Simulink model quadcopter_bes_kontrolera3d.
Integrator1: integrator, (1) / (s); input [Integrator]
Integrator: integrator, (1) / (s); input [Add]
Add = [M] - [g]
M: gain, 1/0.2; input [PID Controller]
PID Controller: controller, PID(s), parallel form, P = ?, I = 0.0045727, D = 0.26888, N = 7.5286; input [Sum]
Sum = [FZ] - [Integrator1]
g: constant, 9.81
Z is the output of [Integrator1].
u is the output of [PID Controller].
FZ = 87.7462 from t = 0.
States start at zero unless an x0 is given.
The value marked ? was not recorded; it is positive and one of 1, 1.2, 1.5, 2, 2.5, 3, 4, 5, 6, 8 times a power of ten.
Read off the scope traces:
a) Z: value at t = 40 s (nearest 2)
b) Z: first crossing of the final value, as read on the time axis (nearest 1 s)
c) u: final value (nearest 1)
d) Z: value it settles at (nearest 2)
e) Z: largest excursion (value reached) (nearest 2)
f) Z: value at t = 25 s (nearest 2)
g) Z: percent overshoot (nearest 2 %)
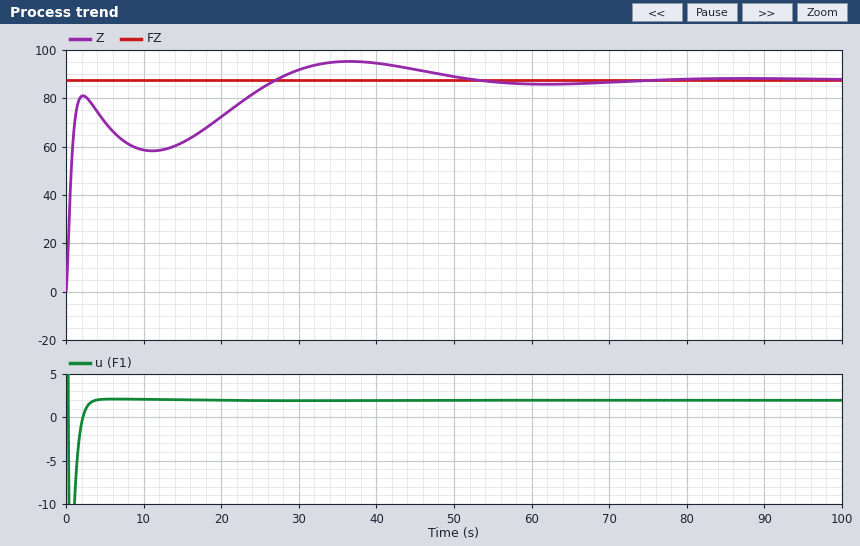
94
27 s
2
88
96
84
8 %
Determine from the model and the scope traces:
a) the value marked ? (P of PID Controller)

0.03
